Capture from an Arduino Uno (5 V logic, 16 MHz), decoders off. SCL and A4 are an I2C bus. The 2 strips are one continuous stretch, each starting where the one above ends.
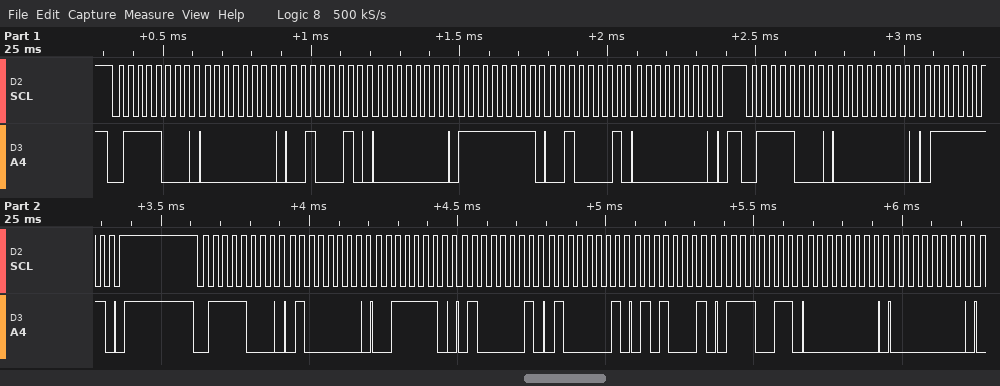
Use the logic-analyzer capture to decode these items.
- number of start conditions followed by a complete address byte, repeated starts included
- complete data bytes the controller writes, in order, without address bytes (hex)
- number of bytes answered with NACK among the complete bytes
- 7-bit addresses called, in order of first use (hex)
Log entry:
3
00 22 00 FF 21 00 00 7F 40 3E 41 41 51 73 00 00
0
0x3C
